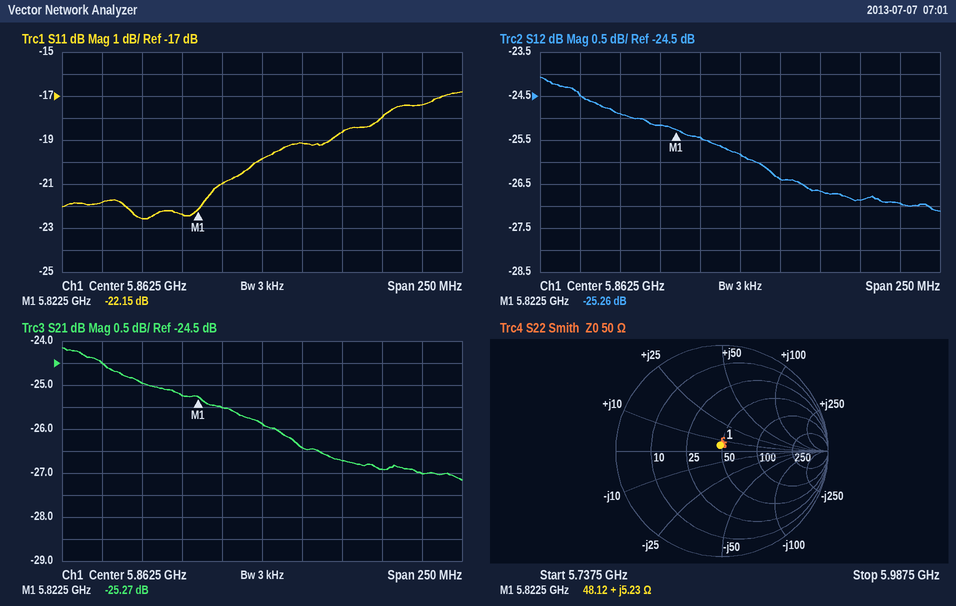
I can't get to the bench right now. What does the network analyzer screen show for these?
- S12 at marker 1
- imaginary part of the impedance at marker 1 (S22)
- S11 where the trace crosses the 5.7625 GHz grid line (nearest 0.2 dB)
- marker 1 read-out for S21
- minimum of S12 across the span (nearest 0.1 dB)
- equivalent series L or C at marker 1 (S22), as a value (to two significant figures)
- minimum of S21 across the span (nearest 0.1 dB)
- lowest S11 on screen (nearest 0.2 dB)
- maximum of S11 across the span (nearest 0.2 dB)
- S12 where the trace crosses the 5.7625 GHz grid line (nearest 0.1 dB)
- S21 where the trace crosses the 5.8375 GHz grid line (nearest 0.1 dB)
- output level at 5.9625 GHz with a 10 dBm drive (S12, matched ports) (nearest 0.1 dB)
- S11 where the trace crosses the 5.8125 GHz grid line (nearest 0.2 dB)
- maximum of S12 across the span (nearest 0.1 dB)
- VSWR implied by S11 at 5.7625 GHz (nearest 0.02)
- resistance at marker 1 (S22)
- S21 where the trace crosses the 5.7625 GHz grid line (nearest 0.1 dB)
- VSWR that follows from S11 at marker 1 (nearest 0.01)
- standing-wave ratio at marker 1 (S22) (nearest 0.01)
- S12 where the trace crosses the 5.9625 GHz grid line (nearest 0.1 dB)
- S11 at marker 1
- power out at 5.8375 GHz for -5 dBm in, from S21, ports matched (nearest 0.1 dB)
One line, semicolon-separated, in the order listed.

-25.26 dB; +5.23 Ω; -21.8 dB; -25.27 dB; -27.1 dB; 140 pH; -27.2 dB; -22.6 dB; -16.8 dB; -24.5 dB; -25.5 dB; -16.9 dBm; -22.4 dB; -24.1 dB; 1.18; 48.12 Ω; -24.5 dB; 1.17; 1.12; -26.9 dB; -22.15 dB; -30.5 dBm
